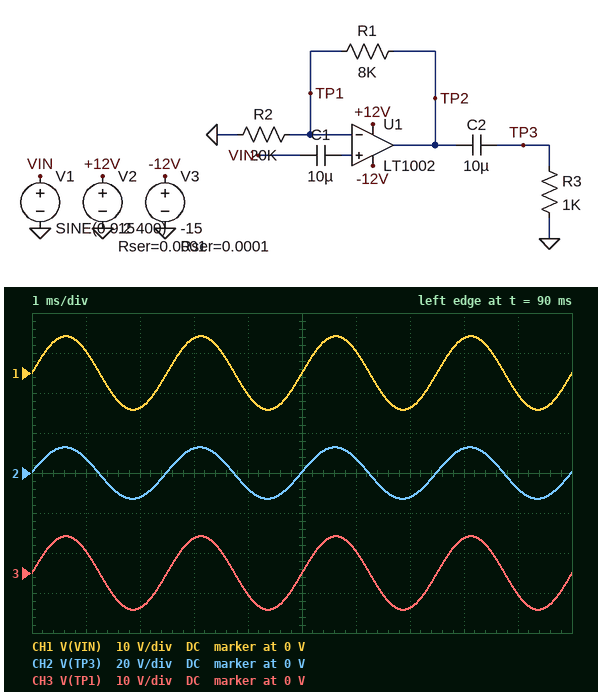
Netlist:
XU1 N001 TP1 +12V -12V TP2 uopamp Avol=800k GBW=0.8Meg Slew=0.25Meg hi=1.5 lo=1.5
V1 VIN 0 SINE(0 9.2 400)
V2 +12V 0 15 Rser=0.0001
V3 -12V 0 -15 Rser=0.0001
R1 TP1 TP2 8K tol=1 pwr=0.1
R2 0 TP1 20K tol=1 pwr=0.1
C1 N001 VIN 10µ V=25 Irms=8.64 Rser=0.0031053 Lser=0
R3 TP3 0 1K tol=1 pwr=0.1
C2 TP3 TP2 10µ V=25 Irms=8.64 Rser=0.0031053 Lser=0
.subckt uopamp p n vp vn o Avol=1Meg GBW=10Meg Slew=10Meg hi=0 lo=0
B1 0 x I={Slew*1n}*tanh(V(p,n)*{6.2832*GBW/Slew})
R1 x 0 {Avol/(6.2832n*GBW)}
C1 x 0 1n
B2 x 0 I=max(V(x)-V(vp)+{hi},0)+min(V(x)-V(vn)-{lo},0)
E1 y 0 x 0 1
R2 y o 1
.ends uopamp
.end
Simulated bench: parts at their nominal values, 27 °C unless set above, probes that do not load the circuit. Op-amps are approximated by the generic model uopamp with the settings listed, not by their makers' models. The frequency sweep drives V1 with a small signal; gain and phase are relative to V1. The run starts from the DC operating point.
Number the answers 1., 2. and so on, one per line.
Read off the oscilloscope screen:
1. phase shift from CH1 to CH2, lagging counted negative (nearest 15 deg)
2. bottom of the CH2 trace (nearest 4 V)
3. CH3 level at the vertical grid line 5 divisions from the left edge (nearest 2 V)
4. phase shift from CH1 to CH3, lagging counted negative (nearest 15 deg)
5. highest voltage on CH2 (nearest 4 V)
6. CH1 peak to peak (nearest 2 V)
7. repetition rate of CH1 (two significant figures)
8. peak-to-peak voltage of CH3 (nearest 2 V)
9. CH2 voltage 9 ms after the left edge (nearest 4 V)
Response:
1. 0 deg
2. -12 V
3. 0 V
4. 0 deg
5. 12 V
6. 18 V
7. 400 Hz
8. 18 V
9. -8 V
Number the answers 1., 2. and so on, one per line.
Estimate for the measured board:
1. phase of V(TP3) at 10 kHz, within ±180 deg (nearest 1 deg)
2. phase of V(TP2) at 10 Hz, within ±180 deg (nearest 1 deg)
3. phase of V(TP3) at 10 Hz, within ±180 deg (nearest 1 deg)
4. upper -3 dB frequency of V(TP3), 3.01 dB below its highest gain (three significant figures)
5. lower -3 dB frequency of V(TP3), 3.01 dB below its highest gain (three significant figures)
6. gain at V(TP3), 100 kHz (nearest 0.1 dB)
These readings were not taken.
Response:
1. -1 deg
2. 0 deg
3. 58 deg
4. 571 kHz
5. 15.9 Hz
6. 2.8 dB
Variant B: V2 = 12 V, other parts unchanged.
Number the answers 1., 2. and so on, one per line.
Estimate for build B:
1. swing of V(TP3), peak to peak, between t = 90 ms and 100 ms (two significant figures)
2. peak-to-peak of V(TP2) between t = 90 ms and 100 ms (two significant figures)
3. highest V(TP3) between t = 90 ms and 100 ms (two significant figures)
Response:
1. 24 V
2. 23 V
3. 11 V
